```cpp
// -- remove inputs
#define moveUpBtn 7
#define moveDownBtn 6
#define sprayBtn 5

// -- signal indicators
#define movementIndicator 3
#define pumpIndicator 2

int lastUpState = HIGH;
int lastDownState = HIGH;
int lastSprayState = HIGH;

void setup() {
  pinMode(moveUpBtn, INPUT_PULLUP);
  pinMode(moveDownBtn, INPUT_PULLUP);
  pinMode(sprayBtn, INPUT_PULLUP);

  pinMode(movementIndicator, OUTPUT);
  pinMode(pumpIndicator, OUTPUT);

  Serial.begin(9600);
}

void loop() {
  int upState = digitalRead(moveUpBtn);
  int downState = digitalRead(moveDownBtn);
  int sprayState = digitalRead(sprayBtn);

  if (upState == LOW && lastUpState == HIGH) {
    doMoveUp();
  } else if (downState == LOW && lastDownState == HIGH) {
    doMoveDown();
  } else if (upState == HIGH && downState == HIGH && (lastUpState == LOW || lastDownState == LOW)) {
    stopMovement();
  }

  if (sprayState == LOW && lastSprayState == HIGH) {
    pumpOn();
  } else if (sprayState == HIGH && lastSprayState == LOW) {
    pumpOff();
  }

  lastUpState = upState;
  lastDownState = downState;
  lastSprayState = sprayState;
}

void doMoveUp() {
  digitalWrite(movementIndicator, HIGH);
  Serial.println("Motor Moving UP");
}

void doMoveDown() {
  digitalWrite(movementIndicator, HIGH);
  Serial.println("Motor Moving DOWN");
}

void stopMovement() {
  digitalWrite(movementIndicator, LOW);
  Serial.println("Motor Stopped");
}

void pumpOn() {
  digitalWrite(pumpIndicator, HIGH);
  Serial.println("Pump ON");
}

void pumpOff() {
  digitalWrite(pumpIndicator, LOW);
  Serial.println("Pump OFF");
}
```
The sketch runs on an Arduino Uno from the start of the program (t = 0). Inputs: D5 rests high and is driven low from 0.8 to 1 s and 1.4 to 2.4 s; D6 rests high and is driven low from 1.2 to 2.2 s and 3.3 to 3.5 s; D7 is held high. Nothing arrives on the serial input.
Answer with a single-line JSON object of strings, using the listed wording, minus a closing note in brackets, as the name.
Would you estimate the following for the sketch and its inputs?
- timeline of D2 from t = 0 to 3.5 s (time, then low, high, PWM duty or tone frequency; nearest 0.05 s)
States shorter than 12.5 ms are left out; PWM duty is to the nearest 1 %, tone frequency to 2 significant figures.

{"timeline of D2 from t = 0 to 3.5 s": "0 s low; 0.8 s high; 1 s low; 1.4 s high; 2.4 s low"}
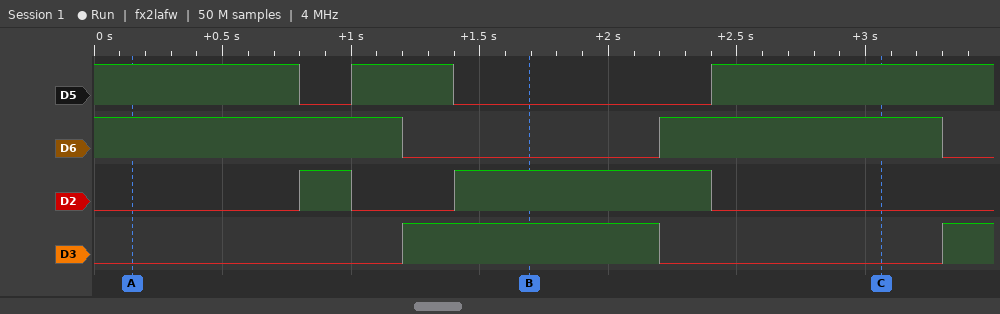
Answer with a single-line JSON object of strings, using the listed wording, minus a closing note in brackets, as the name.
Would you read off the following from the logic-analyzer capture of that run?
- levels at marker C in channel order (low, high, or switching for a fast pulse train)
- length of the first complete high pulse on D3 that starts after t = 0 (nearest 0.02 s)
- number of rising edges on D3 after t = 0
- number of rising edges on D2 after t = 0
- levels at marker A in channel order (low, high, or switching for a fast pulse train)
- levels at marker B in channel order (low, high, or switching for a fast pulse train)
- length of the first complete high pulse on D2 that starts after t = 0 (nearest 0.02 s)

{"levels at marker C in channel order": "D5 high, D6 high, D2 low, D3 low", "length of the first complete high pulse on D3 that starts after t = 0": "1.00 s", "number of rising edges on D3 after t = 0": "2", "number of rising edges on D2 after t = 0": "2", "levels at marker A in channel order": "D5 high, D6 high, D2 low, D3 low", "levels at marker B in channel order": "D5 low, D6 low, D2 high, D3 high", "length of the first complete high pulse on D2 that starts after t = 0": "0.20 s"}
